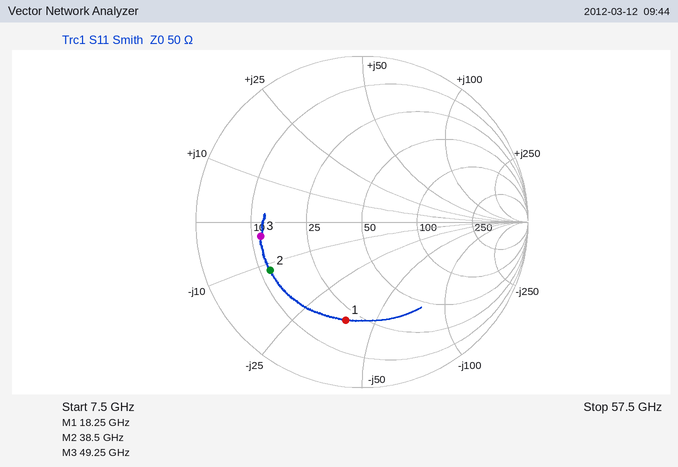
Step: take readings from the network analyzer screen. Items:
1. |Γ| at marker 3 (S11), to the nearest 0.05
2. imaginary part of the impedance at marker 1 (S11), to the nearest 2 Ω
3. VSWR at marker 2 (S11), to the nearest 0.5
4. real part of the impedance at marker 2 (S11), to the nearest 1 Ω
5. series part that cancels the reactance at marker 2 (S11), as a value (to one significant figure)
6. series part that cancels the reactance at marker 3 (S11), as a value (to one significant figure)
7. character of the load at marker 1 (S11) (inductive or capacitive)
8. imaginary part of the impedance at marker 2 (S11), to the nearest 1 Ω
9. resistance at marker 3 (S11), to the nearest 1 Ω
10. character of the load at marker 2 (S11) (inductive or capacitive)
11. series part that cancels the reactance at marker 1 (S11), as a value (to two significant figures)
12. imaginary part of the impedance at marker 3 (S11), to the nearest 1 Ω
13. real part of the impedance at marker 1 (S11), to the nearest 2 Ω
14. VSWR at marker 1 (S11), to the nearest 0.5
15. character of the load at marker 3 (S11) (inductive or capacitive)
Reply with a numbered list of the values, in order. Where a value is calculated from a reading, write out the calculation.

1. 0.60
2. -38 Ω
3. 4.5
4. 12 Ω
5. L = 12 Ω/(2π × 38.5 GHz) ≈ 50 pH
6. L = 3 Ω/(2π × 49.25 GHz) ≈ 10 pH
7. capacitive
8. -12 Ω
9. 12 Ω
10. capacitive
11. L = 38 Ω/(2π × 18.25 GHz) ≈ 331 pH, so 330 pH to two significant figures
12. -3 Ω
13. 20 Ω
14. 4.0
15. capacitive
